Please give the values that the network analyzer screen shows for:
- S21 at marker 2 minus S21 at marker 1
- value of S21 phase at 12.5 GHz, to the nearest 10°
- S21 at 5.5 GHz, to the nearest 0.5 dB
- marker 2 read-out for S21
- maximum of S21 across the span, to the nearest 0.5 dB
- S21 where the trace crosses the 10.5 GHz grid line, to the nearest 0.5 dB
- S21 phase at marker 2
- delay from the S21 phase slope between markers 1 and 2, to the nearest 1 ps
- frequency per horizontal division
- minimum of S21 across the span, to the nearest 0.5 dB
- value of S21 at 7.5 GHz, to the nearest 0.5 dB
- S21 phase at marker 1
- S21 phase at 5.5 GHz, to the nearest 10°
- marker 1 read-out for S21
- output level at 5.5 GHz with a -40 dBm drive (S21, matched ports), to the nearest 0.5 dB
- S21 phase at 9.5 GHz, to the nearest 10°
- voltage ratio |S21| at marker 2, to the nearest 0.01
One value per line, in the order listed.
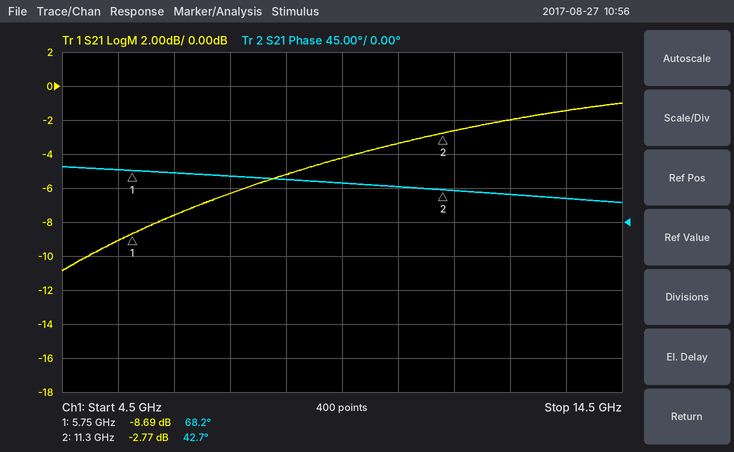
5.92 dB
40°
-9.0 dB
-2.77 dB
-1.0 dB
-3.5 dB
42.7°
13 ps
1 GHz
-11.0 dB
-6.5 dB
68.2°
70°
-8.69 dB
-49.0 dBm
50°
0.73
